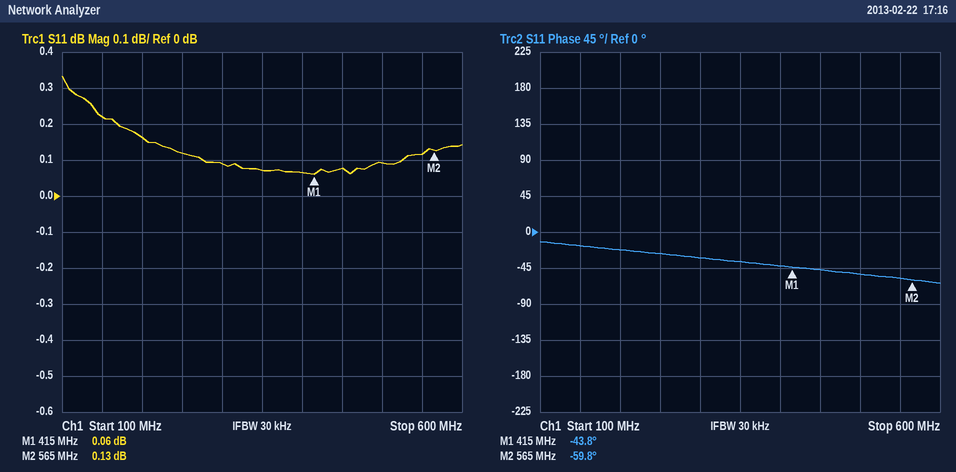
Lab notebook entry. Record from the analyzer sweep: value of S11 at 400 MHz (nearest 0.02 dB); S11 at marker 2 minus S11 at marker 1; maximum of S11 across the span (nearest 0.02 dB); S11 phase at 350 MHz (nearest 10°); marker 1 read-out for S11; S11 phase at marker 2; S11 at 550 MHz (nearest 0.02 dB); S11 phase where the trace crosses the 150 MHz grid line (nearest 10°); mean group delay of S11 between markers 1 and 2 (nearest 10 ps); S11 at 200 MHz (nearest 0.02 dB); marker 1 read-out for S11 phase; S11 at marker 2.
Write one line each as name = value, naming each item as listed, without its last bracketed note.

value of S11 at 400 MHz = 0.06 dB
S11 at marker 2 minus S11 at marker 1 = 0.07 dB
maximum of S11 across the span = 0.34 dB
S11 phase at 350 MHz = -40°
marker 1 read-out for S11 = 0.06 dB
S11 phase at marker 2 = -59.8°
S11 at 550 MHz = 0.12 dB
S11 phase where the trace crosses the 150 MHz grid line = -20°
mean group delay of S11 between markers 1 and 2 = 300 ps
S11 at 200 MHz = 0.16 dB
marker 1 read-out for S11 phase = -43.8°
S11 at marker 2 = 0.13 dB
